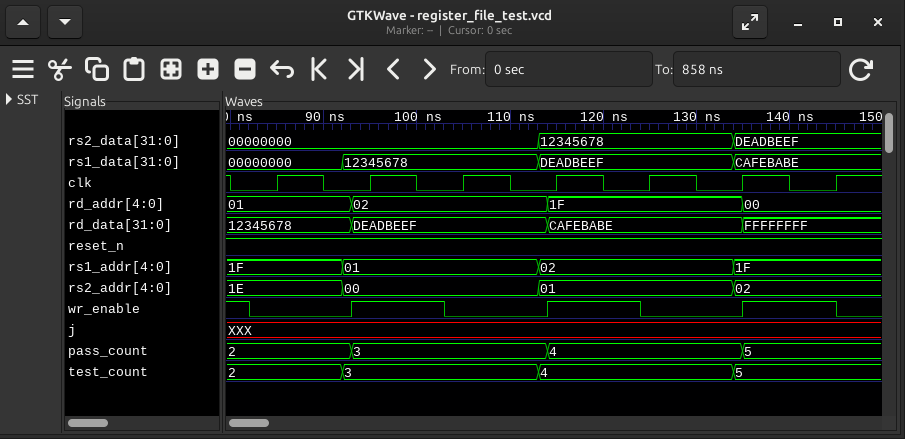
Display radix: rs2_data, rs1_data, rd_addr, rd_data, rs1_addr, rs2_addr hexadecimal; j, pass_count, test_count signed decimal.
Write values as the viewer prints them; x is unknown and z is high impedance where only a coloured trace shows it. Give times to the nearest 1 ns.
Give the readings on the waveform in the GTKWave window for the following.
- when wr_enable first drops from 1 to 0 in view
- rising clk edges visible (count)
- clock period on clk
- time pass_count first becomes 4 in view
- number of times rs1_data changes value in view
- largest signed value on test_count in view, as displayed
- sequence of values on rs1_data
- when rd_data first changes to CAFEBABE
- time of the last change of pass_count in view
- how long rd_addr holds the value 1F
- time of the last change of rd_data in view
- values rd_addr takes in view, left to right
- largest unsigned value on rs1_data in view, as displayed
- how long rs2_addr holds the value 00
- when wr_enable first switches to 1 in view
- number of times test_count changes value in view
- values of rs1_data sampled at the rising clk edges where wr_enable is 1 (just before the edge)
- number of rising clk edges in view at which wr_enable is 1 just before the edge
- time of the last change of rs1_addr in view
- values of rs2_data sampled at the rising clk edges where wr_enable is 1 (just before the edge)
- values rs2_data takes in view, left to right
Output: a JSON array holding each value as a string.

["82 ns", "7", "10 ns", "114 ns", "3", "5", "00000000, 12345678, DEADBEEF, CAFEBABE", "114 ns", "135 ns", "21 ns", "135 ns", "01, 02, 1F, 00", "DEADBEEF", "21 ns", "93 ns", "3", "12345678, DEADBEEF, CAFEBABE", "3", "134 ns", "00000000, 12345678, DEADBEEF", "00000000, 12345678, DEADBEEF"]
